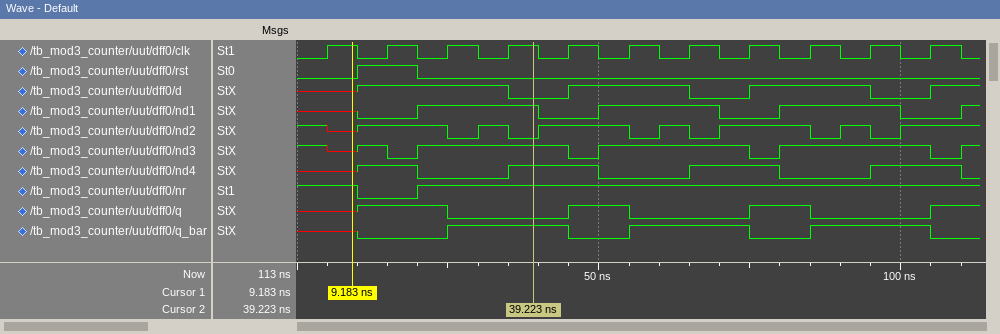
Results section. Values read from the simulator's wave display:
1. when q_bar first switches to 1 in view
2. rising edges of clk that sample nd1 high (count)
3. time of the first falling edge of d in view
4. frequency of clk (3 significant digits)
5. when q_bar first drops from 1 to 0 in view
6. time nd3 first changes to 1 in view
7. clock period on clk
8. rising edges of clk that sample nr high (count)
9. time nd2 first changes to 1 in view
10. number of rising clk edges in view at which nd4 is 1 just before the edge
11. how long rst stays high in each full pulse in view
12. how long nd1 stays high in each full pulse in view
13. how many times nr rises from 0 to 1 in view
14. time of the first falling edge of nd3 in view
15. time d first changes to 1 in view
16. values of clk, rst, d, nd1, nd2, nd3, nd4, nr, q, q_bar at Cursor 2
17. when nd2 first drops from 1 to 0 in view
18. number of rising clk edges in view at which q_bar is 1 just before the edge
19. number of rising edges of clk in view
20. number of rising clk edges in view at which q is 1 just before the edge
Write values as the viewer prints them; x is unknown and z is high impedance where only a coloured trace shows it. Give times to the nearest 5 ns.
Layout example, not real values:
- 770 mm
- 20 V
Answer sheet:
- 25 ns
- 6
- 35 ns
- 100 MHz
- 45 ns
- 10 ns
- 10 ns
- 10
- 10 ns
- 4
- 10 ns
- 20 ns, 20 ns, 20 ns
- 1
- 15 ns
- 10 ns
- clk=1, rst=0, d=0, nd1=1, nd2=0, nd3=1, nd4=1, nr=1, q=0, q_bar=1
- 25 ns
- 6
- 11
- 4
